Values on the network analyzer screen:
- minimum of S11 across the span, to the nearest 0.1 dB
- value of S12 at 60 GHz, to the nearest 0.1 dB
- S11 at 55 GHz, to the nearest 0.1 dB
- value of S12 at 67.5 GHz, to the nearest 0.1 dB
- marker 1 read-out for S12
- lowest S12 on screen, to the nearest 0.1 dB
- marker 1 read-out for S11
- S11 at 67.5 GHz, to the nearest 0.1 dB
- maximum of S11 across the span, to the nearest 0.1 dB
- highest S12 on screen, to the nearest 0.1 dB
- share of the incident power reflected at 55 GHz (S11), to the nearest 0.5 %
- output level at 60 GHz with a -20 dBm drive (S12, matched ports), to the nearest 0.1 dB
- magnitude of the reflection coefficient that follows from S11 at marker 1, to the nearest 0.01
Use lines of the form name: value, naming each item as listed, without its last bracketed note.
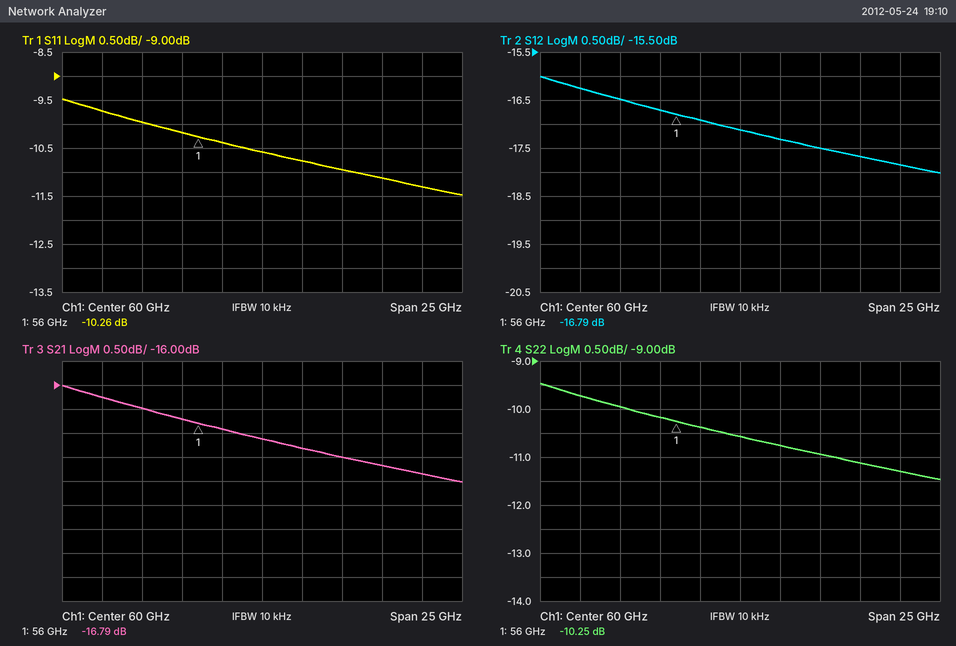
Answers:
minimum of S11 across the span, to the nearest 0.1 dB: -11.5 dB
value of S12 at 60 GHz, to the nearest 0.1 dB: -17.1 dB
S11 at 55 GHz, to the nearest 0.1 dB: -10.2 dB
value of S12 at 67.5 GHz, to the nearest 0.1 dB: -17.7 dB
marker 1 read-out for S12: -16.79 dB
lowest S12 on screen, to the nearest 0.1 dB: -18.0 dB
marker 1 read-out for S11: -10.26 dB
S11 at 67.5 GHz, to the nearest 0.1 dB: -11.1 dB
maximum of S11 across the span, to the nearest 0.1 dB: -9.5 dB
highest S12 on screen, to the nearest 0.1 dB: -16.0 dB
share of the incident power reflected at 55 GHz (S11), to the nearest 0.5 %: 9.5 %
output level at 60 GHz with a -20 dBm drive (S12, matched ports), to the nearest 0.1 dB: -37.1 dBm
magnitude of the reflection coefficient that follows from S11 at marker 1, to the nearest 0.01: 0.31
